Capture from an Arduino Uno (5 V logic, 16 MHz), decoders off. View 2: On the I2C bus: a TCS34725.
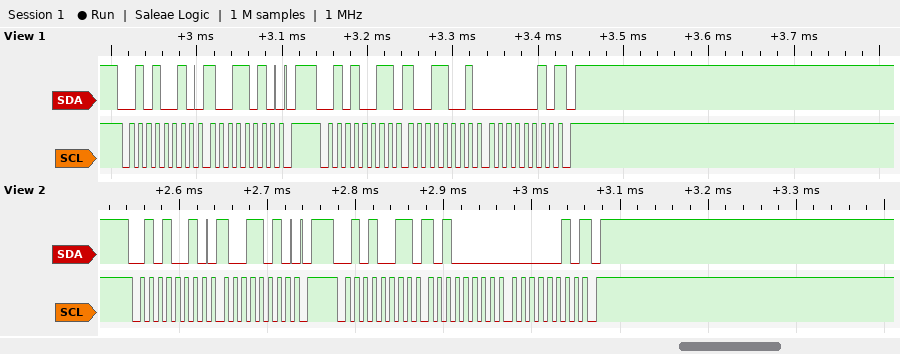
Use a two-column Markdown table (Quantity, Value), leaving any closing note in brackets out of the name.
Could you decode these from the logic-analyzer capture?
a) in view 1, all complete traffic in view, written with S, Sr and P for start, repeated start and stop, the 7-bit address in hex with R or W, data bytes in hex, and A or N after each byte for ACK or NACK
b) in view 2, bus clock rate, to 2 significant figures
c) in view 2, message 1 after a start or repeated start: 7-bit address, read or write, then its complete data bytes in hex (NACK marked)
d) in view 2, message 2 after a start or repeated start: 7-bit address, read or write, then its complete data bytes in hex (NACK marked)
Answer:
| Quantity | Value |
|---|---|
| in view 1, all complete traffic in view, written with S, Sr and P for start, repeated start and stop, the 7-bit address in hex with R or W, data bytes in hex, and A or N after each byte for ACK or NACK | S 29W A 9A A P S 29R A 99 A 02 N P |
| in view 2, bus clock rate, to 2 significant figures | 100 kHz |
| in view 2, message 1 after a start or repeated start: 7-bit address, read or write, then its complete data bytes in hex | 0x29 write: 9A |
| in view 2, message 2 after a start or repeated start: 7-bit address, read or write, then its complete data bytes in hex | 0x29 read: A0 02 NACK |
